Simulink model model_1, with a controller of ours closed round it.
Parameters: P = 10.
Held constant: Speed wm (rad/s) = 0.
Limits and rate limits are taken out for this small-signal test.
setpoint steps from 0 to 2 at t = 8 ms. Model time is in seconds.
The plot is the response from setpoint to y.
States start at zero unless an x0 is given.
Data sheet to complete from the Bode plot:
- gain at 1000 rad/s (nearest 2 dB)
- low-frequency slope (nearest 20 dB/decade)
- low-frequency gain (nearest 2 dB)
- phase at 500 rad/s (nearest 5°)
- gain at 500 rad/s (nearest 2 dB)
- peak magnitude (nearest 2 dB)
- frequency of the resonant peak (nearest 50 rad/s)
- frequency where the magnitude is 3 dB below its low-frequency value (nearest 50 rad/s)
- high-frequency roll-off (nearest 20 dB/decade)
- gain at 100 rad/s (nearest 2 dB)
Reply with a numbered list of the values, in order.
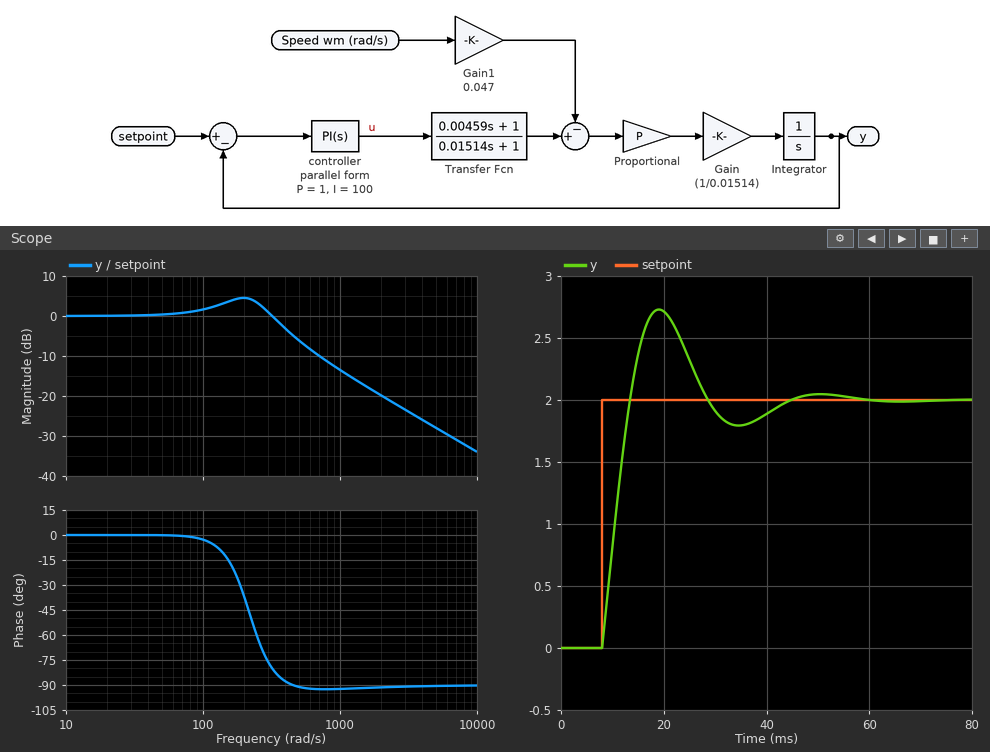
1. -14 dB
2. 0 dB/decade
3. 0 dB
4. -90°
5. -6 dB
6. 4 dB
7. 200 rad/s
8. 400 rad/s
9. -20 dB/decade
10. 2 dB
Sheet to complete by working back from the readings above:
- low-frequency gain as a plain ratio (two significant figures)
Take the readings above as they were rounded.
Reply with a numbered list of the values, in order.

1. 1.0
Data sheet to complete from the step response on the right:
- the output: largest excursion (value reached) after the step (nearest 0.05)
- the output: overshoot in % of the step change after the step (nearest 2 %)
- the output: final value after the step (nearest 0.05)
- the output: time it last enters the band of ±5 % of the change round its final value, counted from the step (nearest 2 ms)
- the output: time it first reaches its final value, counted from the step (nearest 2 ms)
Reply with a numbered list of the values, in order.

1. 2.75
2. 36 %
3. 2.00
4. 32 ms
5. 6 ms
